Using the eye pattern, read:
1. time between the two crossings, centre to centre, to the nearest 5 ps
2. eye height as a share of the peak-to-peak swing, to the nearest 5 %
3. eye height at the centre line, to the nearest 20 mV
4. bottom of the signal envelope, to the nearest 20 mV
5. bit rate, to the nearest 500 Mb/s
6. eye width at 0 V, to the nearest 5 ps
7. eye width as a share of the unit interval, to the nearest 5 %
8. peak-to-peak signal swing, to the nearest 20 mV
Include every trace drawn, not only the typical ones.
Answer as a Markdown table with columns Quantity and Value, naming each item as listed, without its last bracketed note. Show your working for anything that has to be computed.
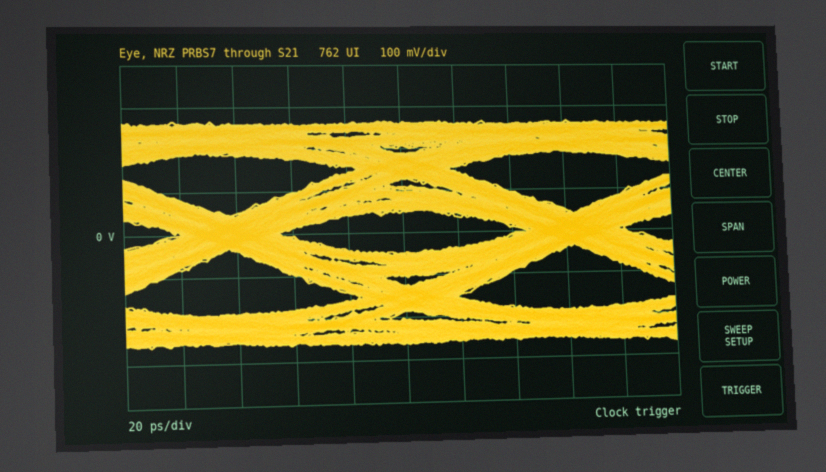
| Quantity | Value |
|---|---|
| time between the two crossings, centre to centre, to the nearest 5 ps | 125 ps |
| eye height as a share of the peak-to-peak swing, to the nearest 5 % | 100 mV / 540 mV ≈ 18.5 %, so 20 % to the nearest 5 % |
| eye height at the centre line, to the nearest 20 mV | 100 mV |
| bottom of the signal envelope, to the nearest 20 mV | -260 mV |
| bit rate, to the nearest 500 Mb/s | 8.0 Gb/s |
| eye width at 0 V, to the nearest 5 ps | 90 ps |
| eye width as a share of the unit interval, to the nearest 5 % | 90 ps / 125 ps ≈ 72.0 %, so 70 % to the nearest 5 % |
| peak-to-peak signal swing, to the nearest 20 mV | 540 mV |
